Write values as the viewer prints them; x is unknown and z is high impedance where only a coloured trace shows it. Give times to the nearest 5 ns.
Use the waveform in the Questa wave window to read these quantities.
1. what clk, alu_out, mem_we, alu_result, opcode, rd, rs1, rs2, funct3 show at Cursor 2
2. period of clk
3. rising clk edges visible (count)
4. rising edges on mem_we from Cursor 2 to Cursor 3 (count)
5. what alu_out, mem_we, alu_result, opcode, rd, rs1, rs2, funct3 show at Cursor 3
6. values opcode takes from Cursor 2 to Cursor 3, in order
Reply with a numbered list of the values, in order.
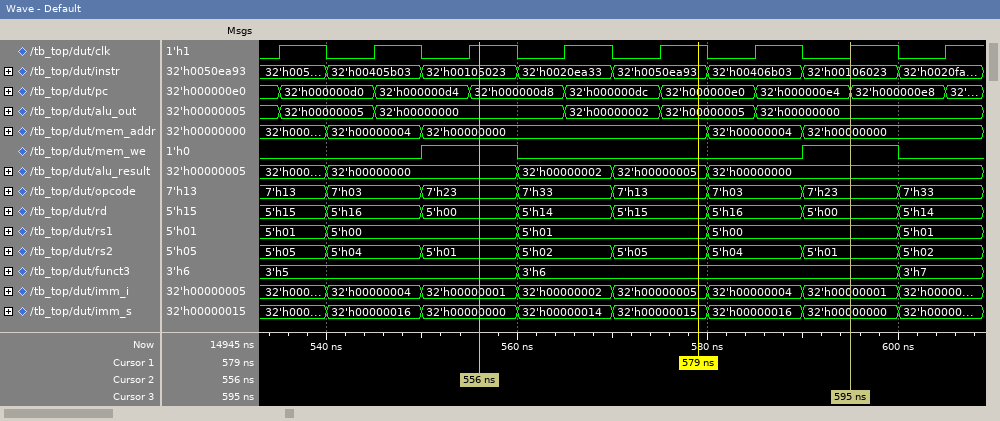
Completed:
1. clk=1, alu_out=32'h00000000, mem_we=1, alu_result=32'h00000000, opcode=7'h23, rd=5'h00, rs1=5'h00, rs2=5'h01, funct3=3'h5
2. 10 ns
3. 8
4. 1
5. alu_out=32'h00000000, mem_we=1, alu_result=32'h00000000, opcode=7'h23, rd=5'h00, rs1=5'h00, rs2=5'h01, funct3=3'h6
6. 7'h23, 7'h33, 7'h13, 7'h03, 7'h23
